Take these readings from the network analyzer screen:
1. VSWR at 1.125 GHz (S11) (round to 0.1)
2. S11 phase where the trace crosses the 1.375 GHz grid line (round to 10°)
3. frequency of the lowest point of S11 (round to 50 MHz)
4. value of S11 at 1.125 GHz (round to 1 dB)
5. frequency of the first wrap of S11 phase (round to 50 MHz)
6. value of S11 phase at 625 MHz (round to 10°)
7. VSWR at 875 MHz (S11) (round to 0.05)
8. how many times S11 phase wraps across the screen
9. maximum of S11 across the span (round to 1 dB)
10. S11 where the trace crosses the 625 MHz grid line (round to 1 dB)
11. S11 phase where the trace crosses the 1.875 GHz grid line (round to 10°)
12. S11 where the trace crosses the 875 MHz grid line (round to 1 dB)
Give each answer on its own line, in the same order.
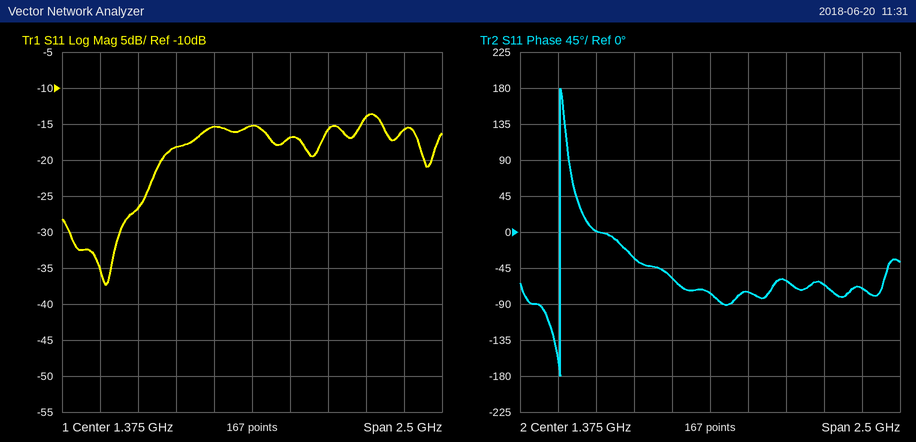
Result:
1.4
-80°
400 MHz
-15 dB
400 MHz
0°
1.30
1
-14 dB
-27 dB
-60°
-18 dB
